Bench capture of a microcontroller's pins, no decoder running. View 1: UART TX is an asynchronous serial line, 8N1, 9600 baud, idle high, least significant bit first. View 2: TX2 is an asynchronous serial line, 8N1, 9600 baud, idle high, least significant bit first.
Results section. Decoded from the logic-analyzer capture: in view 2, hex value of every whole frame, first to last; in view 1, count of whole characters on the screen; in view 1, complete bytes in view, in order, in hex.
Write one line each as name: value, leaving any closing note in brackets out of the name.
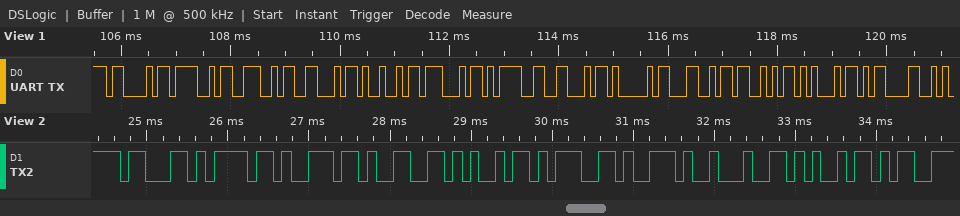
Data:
in view 2, hex value of every whole frame, first to last: 0x63 0x6F 0x6E 0x66 0x69 0x67 0x2E 0x64 0x69
in view 1, count of whole characters on the screen: 13
in view 1, complete bytes in view, in order, in hex: 43 4F 4E 46 49 47 3D 46 41 4C 53 45 0D
